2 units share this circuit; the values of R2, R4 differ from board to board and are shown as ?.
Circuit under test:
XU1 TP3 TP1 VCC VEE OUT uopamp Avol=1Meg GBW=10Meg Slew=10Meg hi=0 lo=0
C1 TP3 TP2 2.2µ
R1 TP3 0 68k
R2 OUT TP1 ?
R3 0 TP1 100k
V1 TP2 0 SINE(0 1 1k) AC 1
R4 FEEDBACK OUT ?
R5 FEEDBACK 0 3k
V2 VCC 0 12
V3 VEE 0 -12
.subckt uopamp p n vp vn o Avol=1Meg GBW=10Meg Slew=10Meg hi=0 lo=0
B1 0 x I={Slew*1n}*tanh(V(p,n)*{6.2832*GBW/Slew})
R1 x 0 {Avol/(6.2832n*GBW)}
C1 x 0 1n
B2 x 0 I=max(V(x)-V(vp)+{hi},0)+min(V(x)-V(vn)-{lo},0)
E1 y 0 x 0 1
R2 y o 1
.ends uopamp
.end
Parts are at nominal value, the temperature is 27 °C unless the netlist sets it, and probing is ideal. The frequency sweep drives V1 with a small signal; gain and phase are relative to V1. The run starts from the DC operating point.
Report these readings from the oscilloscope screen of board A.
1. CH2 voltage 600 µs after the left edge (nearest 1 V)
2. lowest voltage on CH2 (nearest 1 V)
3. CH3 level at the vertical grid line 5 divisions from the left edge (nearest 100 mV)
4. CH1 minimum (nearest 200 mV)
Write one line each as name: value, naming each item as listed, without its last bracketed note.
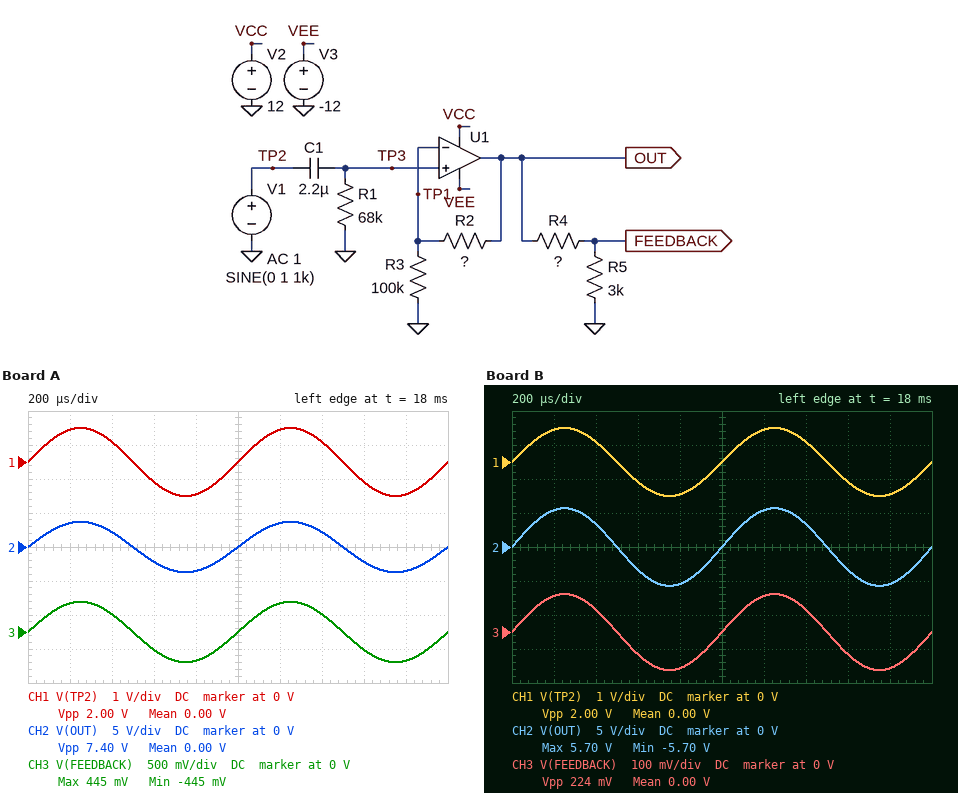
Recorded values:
CH2 voltage 600 µs after the left edge: -2 V
lowest voltage on CH2: -4 V
CH3 level at the vertical grid line 5 divisions from the left edge: 0 V
CH1 minimum: -1.0 V
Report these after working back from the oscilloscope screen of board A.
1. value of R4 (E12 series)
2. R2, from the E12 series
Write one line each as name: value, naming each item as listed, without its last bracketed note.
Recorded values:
value of R4: 22 kΩ
R2, from the E12 series: 270 kΩ
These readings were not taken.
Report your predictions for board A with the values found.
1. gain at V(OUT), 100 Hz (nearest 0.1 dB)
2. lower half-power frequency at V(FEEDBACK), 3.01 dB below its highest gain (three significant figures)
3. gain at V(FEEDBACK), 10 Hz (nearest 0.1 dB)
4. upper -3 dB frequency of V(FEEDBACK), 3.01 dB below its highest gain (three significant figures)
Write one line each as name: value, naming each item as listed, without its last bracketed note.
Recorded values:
gain at V(OUT), 100 Hz: 11.4 dB
lower half-power frequency at V(FEEDBACK), 3.01 dB below its highest gain: 1.06 Hz
gain at V(FEEDBACK), 10 Hz: -7.1 dB
upper -3 dB frequency of V(FEEDBACK), 3.01 dB below its highest gain: 2.70 MHz
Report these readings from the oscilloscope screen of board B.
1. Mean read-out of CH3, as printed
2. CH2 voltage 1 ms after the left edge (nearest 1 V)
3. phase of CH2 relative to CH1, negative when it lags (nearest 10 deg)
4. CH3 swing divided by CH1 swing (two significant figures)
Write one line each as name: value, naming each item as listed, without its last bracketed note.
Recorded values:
Mean read-out of CH3, as printed: 0.00 V
CH2 voltage 1 ms after the left edge: 0 V
phase of CH2 relative to CH1, negative when it lags: 0 deg
CH3 swing divided by CH1 swing: 0.11
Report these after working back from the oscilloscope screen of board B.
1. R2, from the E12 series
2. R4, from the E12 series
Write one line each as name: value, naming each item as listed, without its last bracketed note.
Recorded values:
R2, from the E12 series: 470 kΩ
R4, from the E12 series: 150 kΩ
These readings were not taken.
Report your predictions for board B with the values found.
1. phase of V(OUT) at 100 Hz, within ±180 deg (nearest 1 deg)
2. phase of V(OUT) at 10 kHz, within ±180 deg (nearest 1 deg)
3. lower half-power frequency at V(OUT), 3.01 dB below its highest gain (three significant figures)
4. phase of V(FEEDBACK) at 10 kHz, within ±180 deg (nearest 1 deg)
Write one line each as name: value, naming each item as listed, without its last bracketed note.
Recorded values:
phase of V(OUT) at 100 Hz, within ±180 deg: 1 deg
phase of V(OUT) at 10 kHz, within ±180 deg: 0 deg
lower half-power frequency at V(OUT), 3.01 dB below its highest gain: 1.06 Hz
phase of V(FEEDBACK) at 10 kHz, within ±180 deg: 0 deg
